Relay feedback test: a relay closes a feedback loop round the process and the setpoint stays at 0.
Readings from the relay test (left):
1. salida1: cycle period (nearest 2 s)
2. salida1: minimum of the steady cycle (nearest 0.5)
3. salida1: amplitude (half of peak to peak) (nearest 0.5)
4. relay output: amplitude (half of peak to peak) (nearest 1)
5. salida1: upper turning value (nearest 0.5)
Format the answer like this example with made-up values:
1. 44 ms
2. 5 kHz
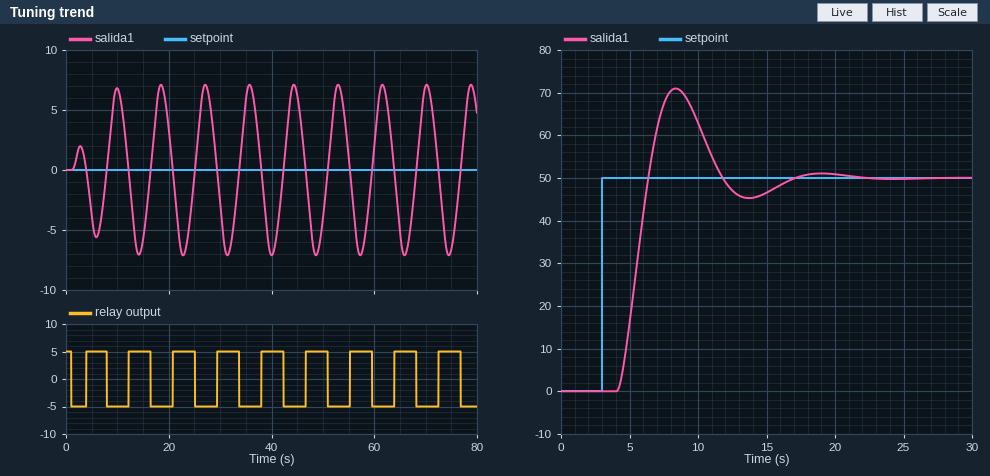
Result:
1. 8 s
2. -7.0
3. 7.0
4. 5
5. 7.0
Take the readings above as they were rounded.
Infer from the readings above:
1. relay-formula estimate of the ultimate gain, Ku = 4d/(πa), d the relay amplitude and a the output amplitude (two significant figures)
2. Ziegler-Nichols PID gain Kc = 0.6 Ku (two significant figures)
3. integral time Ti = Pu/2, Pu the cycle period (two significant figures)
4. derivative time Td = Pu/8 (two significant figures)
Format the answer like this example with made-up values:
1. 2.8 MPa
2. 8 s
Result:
1. 0.91
2. 0.55
3. 4.0 s
4. 1.0 s
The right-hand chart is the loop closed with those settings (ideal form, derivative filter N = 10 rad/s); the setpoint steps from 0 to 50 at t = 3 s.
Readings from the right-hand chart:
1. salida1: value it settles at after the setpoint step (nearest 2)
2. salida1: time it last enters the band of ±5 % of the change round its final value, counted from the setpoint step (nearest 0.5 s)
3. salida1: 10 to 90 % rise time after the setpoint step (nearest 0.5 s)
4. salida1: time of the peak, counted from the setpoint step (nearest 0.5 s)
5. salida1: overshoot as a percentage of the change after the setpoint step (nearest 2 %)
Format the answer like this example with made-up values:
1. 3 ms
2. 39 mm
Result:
1. 50
2. 12.5 s
3. 1.5 s
4. 5.5 s
5. 42 %
